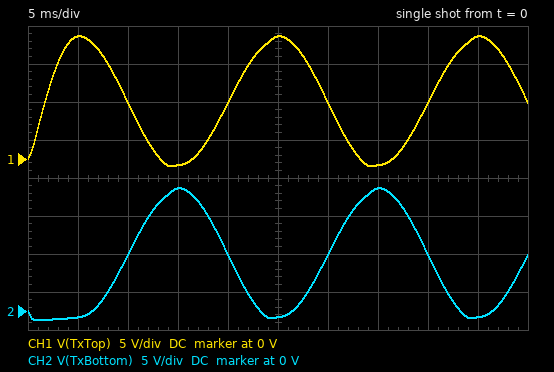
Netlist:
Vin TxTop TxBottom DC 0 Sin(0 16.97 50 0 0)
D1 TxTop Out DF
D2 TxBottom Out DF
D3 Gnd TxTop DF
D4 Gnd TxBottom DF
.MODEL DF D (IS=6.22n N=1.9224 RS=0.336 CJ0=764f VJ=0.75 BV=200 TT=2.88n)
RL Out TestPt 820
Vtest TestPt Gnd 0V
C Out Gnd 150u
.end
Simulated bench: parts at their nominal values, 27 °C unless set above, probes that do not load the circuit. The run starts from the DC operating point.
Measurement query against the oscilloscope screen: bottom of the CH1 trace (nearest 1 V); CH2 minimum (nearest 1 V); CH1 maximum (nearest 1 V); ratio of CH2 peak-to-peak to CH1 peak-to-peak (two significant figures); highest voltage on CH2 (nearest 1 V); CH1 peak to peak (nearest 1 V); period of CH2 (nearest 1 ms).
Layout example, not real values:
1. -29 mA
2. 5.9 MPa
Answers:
1. -1 V
2. -1 V
3. 16 V
4. 1.0
5. 16 V
6. 17 V
7. 20 ms
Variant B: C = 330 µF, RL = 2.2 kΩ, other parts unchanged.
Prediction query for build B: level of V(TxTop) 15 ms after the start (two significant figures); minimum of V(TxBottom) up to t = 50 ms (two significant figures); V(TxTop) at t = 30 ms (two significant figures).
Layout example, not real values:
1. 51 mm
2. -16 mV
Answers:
1. -860 mV
2. -1.5 V
3. 7.6 V
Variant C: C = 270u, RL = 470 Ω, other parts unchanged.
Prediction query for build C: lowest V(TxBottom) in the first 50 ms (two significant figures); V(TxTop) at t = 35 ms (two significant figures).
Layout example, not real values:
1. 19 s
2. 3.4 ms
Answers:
1. -1.4 V
2. -900 mV
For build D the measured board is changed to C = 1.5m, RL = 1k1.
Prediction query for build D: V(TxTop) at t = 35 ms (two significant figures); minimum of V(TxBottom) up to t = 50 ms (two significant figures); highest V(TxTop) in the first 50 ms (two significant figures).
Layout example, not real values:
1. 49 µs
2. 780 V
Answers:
1. -970 mV
2. -3.0 V
3. 16 V
